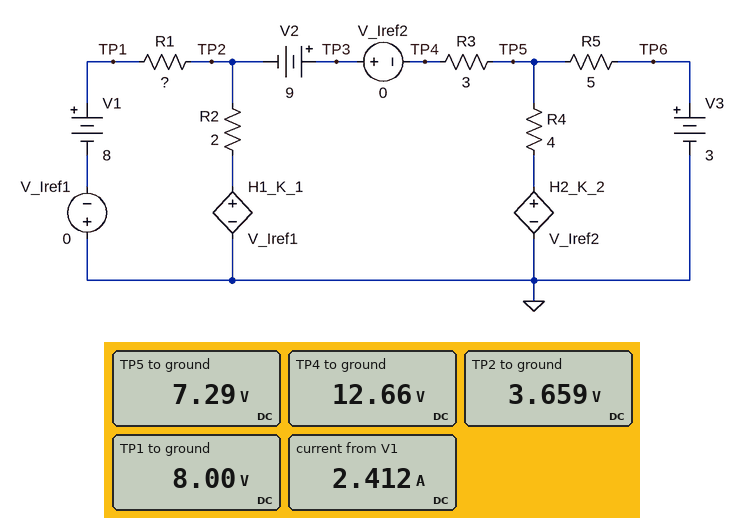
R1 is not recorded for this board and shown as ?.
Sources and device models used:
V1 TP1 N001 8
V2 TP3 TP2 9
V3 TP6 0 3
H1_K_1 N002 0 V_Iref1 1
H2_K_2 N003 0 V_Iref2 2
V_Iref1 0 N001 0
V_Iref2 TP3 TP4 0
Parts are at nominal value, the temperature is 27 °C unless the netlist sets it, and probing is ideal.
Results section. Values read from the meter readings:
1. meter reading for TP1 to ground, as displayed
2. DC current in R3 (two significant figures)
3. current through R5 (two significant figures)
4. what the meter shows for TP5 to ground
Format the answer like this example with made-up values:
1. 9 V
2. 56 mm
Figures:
1. 8.00 V
2. 1.8 A
3. 860 mA
4. 7.29 V
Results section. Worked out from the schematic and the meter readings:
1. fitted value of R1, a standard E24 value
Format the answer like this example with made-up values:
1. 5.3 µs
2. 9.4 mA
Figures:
1. 1.8 Ω
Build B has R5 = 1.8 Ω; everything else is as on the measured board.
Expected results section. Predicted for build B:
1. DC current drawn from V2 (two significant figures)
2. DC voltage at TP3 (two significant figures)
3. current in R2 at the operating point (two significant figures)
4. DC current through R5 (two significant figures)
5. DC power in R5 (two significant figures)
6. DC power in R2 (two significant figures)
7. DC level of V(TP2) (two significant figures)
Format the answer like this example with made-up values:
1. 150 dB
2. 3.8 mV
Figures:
1. 2.1 A
2. 12 V
3. 430 mA
4. 1.7 A
5. 5.1 W
6. 360 mW
7. 3.4 V
